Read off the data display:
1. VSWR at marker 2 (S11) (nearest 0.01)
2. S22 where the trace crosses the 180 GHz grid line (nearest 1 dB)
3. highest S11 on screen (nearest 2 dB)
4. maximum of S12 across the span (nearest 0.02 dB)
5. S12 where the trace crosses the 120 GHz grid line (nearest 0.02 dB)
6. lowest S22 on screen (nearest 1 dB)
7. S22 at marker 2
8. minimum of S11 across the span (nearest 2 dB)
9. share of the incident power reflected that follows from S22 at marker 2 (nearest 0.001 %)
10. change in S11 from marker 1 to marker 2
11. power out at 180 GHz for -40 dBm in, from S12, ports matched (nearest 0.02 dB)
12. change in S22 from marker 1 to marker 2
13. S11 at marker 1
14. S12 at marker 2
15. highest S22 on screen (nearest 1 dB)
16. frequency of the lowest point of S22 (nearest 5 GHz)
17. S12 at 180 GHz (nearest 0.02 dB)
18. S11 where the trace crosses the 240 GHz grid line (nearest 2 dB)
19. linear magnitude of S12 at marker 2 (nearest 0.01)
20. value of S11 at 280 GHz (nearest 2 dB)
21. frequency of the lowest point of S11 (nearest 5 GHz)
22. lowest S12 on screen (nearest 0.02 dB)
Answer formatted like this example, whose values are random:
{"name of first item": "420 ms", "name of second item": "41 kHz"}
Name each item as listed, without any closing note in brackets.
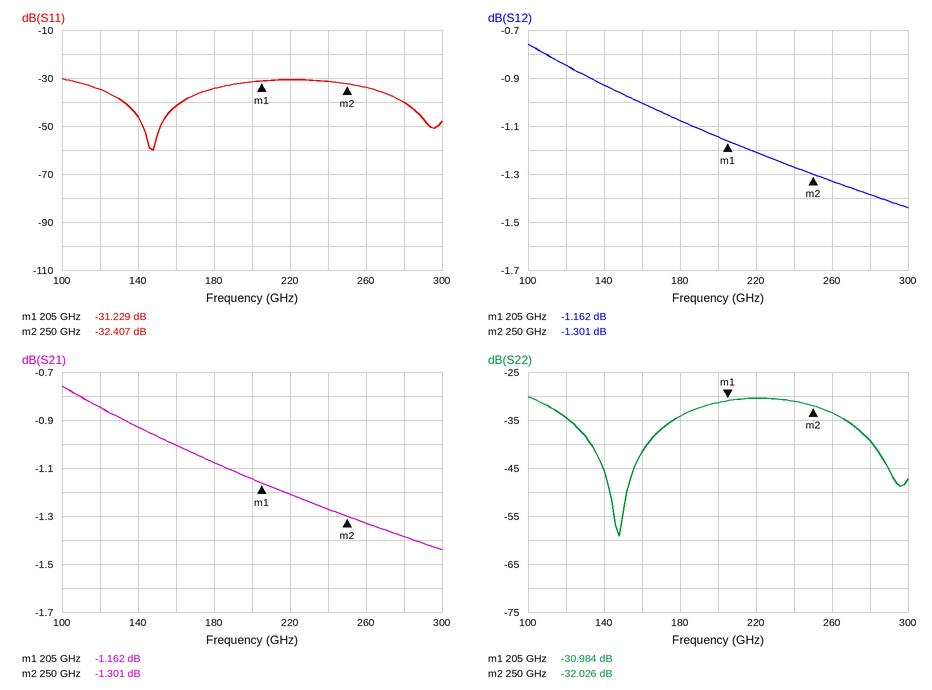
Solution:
{"VSWR at marker 2 (S11)": "1.05", "S22 where the trace crosses the 180 GHz grid line": "-34 dB", "highest S11 on screen": "-30 dB", "maximum of S12 across the span": "-0.76 dB", "S12 where the trace crosses the 120 GHz grid line": "-0.84 dB", "lowest S22 on screen": "-59 dB", "S22 at marker 2": "-32.026 dB", "minimum of S11 across the span": "-60 dB", "share of the incident power reflected that follows from S22 at marker 2": "0.063 %", "change in S11 from marker 1 to marker 2": "-1.178 dB", "power out at 180 GHz for -40 dBm in, from S12, ports matched": "-41.08 dBm", "change in S22 from marker 1 to marker 2": "-1.042 dB", "S11 at marker 1": "-31.229 dB", "S12 at marker 2": "-1.301 dB", "highest S22 on screen": "-30 dB", "frequency of the lowest point of S22": "150 GHz", "S12 at 180 GHz": "-1.08 dB", "S11 where the trace crosses the 240 GHz grid line": "-32 dB", "linear magnitude of S12 at marker 2": "0.86", "value of S11 at 280 GHz": "-40 dB", "frequency of the lowest point of S11": "150 GHz", "lowest S12 on screen": "-1.44 dB"}
